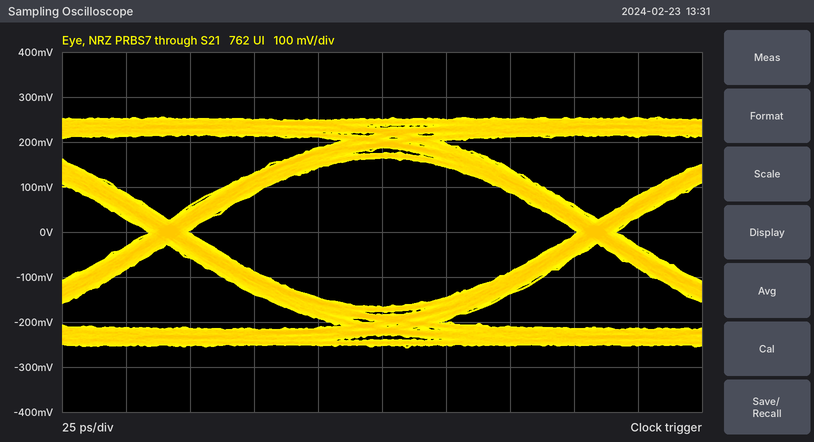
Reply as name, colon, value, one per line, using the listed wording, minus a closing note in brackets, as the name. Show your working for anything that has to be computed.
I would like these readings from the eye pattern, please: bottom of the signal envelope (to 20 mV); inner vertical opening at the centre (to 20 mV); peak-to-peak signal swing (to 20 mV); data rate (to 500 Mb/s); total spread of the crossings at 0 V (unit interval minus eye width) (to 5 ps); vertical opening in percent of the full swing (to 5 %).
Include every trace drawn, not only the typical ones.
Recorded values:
bottom of the signal envelope: -260 mV
inner vertical opening at the centre: 340 mV
peak-to-peak signal swing: 520 mV
data rate: 6.0 Gb/s
total spread of the crossings at 0 V (unit interval minus eye width): 15 ps
vertical opening in percent of the full swing: 340 mV / 520 mV ≈ 65 %
